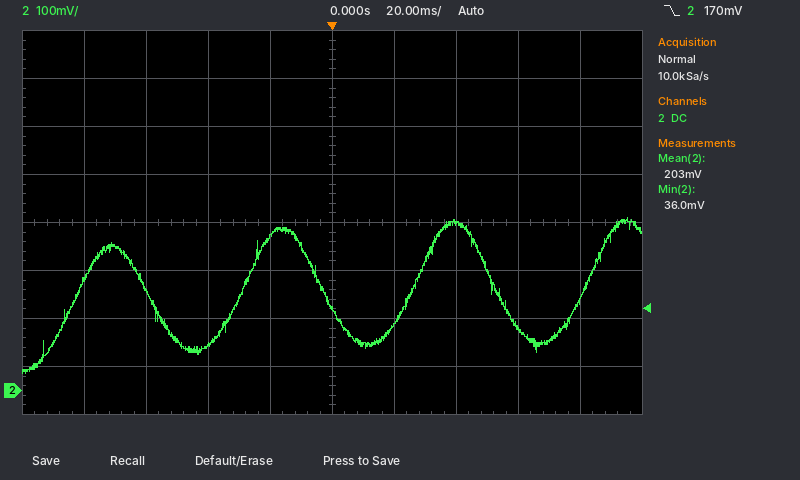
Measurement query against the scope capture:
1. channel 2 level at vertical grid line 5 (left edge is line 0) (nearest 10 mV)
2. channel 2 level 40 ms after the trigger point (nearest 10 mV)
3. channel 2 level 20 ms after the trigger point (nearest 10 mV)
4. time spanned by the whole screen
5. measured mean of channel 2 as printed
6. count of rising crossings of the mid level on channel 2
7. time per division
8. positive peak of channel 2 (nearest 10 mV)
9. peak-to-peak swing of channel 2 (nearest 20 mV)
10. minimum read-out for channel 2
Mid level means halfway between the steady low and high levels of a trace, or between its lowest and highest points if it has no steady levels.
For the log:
170 mV
350 mV
140 mV
200 ms
203 mV
4
20 ms
360 mV
320 mV
36.0 mV
